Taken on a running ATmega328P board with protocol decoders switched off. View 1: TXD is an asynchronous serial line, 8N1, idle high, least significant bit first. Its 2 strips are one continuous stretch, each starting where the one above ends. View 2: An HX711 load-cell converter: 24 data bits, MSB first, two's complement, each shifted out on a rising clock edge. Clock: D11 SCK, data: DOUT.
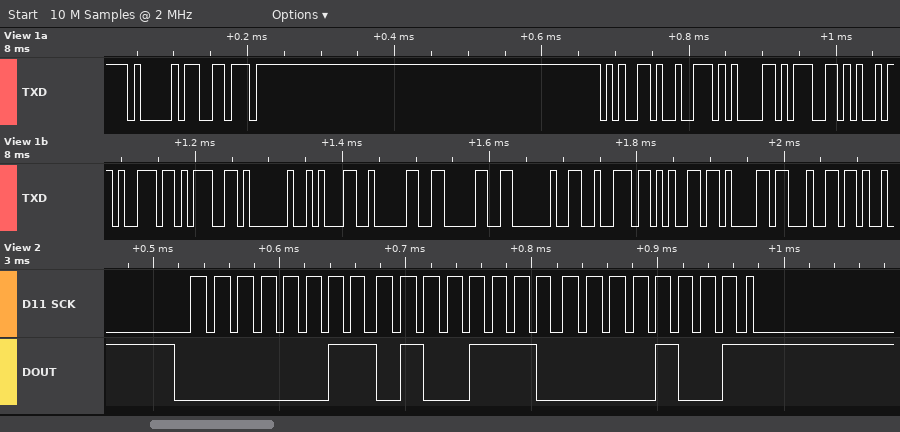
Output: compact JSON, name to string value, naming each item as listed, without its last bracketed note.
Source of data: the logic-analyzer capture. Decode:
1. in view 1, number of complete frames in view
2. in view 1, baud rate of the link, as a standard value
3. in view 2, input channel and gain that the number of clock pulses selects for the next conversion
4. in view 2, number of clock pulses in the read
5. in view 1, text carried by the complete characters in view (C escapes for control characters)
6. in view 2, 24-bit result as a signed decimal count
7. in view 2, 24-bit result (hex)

{"in view 1, number of complete frames in view": "18", "in view 1, baud rate of the link, as a standard value": "115200 baud", "in view 2, input channel and gain that the number of clock pulses selects for the next conversion": "channel A, gain 128", "in view 2, number of clock pulses in the read": "25", "in view 1, text carried by the complete characters in view": "\"Averaging 100 read\"", "in view 2, 24-bit result as a signed decimal count": "216585", "in view 2, 24-bit result": "0x034E09"}
